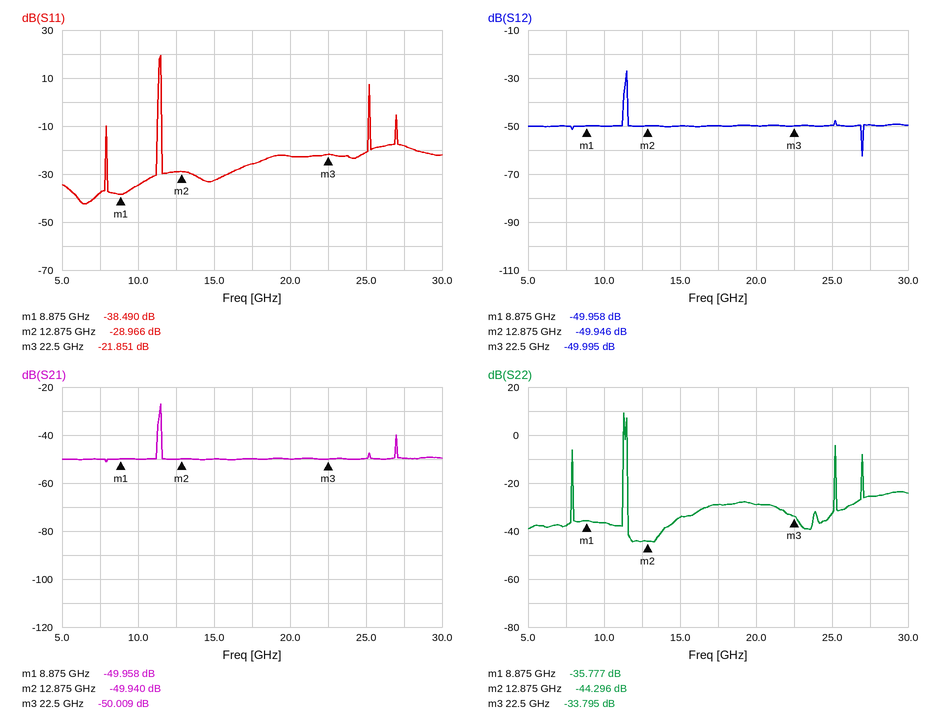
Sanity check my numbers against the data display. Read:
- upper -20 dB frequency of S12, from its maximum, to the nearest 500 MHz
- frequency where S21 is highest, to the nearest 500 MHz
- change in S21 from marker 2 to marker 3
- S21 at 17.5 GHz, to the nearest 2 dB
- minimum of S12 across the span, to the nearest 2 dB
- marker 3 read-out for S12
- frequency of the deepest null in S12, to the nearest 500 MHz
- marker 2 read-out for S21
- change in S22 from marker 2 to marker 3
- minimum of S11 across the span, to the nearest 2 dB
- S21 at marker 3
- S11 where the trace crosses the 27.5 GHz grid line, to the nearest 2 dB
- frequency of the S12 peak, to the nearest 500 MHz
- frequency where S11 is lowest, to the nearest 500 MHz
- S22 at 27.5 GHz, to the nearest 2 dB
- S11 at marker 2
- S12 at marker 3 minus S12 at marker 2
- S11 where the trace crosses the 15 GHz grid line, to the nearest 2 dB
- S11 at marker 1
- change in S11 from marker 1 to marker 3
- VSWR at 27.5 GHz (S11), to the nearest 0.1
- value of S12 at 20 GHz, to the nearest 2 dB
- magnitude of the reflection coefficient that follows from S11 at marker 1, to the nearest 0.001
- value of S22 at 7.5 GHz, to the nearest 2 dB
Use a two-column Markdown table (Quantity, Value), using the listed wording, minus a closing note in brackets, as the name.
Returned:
| Quantity | Value |
|---|---|
| upper -20 dB frequency of S12, from its maximum, to the nearest 500 MHz | 11.5 GHz |
| frequency where S21 is highest, to the nearest 500 MHz | 11.5 GHz |
| change in S21 from marker 2 to marker 3 | -0.069 dB |
| S21 at 17.5 GHz, to the nearest 2 dB | -50 dB |
| minimum of S12 across the span, to the nearest 2 dB | -62 dB |
| marker 3 read-out for S12 | -49.995 dB |
| frequency of the deepest null in S12, to the nearest 500 MHz | 27.0 GHz |
| marker 2 read-out for S21 | -49.940 dB |
| change in S22 from marker 2 to marker 3 | 10.501 dB |
| minimum of S11 across the span, to the nearest 2 dB | -42 dB |
| S21 at marker 3 | -50.009 dB |
| S11 where the trace crosses the 27.5 GHz grid line, to the nearest 2 dB | -18 dB |
| frequency of the S12 peak, to the nearest 500 MHz | 11.5 GHz |
| frequency where S11 is lowest, to the nearest 500 MHz | 6.5 GHz |
| S22 at 27.5 GHz, to the nearest 2 dB | -26 dB |
| S11 at marker 2 | -28.966 dB |
| S12 at marker 3 minus S12 at marker 2 | -0.049 dB |
| S11 where the trace crosses the 15 GHz grid line, to the nearest 2 dB | -32 dB |
| S11 at marker 1 | -38.490 dB |
| change in S11 from marker 1 to marker 3 | 16.639 dB |
| VSWR at 27.5 GHz (S11), to the nearest 0.1 | 1.3 |
| value of S12 at 20 GHz, to the nearest 2 dB | -50 dB |
| magnitude of the reflection coefficient that follows from S11 at marker 1, to the nearest 0.001 | 0.012 |
| value of S22 at 7.5 GHz, to the nearest 2 dB | -38 dB |
